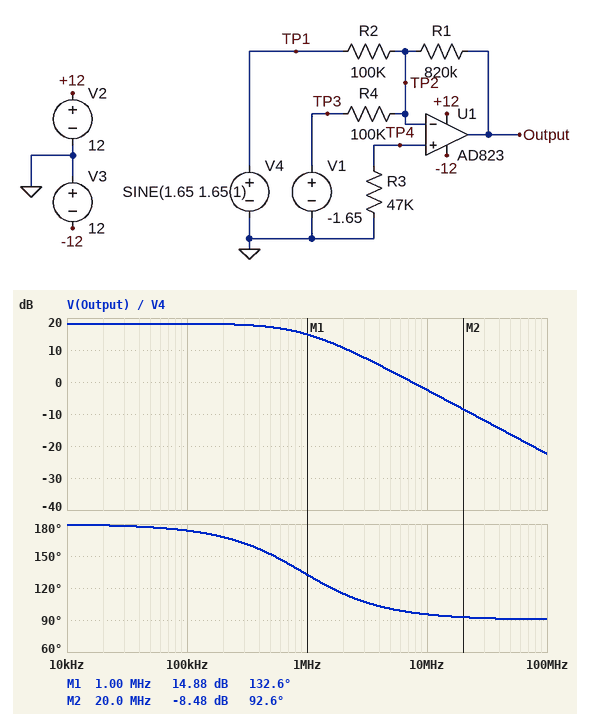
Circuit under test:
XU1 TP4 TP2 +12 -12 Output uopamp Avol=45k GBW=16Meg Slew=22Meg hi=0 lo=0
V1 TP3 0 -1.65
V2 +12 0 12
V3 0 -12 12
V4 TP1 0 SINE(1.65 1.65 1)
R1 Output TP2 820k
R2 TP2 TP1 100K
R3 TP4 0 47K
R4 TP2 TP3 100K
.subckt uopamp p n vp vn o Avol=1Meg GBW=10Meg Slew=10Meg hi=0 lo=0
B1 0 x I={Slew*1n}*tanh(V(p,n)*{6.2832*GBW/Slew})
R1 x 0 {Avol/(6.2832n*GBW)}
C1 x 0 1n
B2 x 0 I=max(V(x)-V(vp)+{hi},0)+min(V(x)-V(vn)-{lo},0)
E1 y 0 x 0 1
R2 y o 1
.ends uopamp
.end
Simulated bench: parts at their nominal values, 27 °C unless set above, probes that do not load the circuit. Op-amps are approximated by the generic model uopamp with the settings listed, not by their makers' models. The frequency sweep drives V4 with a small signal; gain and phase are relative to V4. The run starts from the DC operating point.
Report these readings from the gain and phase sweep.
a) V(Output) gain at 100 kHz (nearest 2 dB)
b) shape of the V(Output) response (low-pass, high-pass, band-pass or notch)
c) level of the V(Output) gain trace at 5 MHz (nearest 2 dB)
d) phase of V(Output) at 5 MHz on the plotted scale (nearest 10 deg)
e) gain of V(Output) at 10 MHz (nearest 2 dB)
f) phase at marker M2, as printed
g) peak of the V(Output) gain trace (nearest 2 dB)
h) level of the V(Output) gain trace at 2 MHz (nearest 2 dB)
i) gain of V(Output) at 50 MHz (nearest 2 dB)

18 dB
low-pass
4 dB
100 deg
-2 dB
92.6 deg
18 dB
10 dB
-16 dB
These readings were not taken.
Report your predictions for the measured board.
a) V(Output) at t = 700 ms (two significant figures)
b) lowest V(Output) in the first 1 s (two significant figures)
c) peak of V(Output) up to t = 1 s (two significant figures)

12 V
-12 V
12 V
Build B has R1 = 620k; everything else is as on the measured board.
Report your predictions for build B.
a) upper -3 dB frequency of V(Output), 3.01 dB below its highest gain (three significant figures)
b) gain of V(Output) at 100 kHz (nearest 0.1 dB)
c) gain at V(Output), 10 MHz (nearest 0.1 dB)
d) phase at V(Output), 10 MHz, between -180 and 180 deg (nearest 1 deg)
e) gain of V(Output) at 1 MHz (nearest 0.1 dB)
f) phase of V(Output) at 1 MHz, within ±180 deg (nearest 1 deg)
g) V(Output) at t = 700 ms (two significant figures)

1.19 MHz
15.8 dB
-2.7 dB
97 deg
13.5 dB
140 deg
9.7 V
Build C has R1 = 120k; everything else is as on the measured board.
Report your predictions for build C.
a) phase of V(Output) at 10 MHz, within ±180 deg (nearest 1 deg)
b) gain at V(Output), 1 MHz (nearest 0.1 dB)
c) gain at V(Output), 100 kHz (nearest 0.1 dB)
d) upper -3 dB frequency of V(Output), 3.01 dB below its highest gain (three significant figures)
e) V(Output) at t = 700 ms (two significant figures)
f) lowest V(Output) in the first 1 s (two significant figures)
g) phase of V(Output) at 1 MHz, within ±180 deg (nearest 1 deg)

115 deg
1.4 dB
1.6 dB
4.71 MHz
1.9 V
-2.0 V
168 deg
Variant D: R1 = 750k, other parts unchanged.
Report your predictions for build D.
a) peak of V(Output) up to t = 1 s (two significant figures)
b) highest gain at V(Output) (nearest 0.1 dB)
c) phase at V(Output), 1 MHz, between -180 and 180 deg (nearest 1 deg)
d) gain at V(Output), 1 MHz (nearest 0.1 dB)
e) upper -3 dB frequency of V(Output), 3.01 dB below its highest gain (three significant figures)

12 V
17.5 dB
135 deg
14.5 dB
1.00 MHz
